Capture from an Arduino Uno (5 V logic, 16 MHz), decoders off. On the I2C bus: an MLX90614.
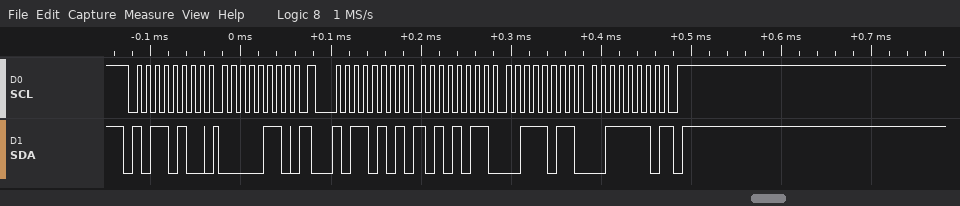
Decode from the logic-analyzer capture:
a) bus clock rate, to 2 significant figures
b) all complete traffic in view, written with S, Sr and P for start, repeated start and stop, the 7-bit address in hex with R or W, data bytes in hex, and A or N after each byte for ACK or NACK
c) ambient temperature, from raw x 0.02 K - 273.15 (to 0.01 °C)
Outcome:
100 kHz
S 5AW A 06 A Sr 5AR A AB A 3B A 3E N P
32.35 °C
